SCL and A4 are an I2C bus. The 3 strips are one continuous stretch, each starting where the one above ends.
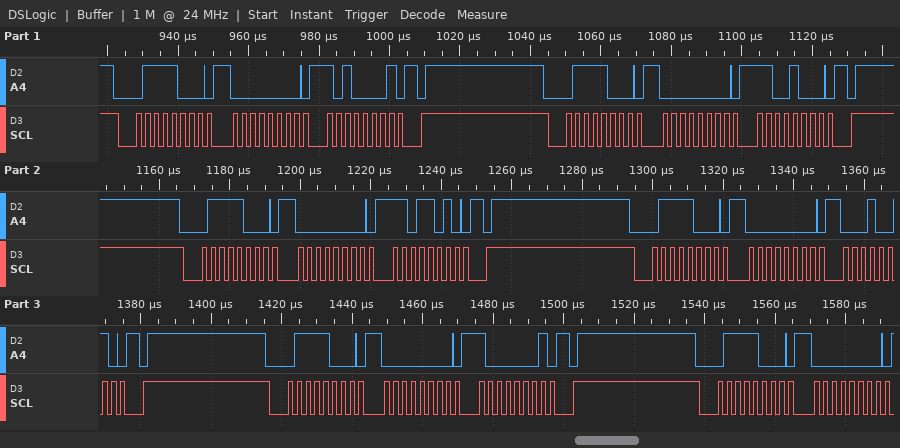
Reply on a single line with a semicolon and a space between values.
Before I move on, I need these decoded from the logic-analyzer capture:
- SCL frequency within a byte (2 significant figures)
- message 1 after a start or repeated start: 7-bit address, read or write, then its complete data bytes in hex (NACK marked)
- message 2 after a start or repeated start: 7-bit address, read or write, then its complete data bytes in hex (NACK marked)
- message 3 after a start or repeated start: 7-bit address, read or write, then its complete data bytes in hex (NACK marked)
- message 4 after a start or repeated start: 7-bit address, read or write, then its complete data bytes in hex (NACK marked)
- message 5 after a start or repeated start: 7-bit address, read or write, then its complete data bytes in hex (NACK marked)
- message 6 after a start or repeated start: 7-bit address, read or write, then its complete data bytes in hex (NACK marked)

400 kHz; 0x3C write: 00 A1; 0x3C write: 00 C8; 0x3C write: 00 DA; 0x3C write: 00 12; 0x3C write: 00 81; 0x3C write: 00
